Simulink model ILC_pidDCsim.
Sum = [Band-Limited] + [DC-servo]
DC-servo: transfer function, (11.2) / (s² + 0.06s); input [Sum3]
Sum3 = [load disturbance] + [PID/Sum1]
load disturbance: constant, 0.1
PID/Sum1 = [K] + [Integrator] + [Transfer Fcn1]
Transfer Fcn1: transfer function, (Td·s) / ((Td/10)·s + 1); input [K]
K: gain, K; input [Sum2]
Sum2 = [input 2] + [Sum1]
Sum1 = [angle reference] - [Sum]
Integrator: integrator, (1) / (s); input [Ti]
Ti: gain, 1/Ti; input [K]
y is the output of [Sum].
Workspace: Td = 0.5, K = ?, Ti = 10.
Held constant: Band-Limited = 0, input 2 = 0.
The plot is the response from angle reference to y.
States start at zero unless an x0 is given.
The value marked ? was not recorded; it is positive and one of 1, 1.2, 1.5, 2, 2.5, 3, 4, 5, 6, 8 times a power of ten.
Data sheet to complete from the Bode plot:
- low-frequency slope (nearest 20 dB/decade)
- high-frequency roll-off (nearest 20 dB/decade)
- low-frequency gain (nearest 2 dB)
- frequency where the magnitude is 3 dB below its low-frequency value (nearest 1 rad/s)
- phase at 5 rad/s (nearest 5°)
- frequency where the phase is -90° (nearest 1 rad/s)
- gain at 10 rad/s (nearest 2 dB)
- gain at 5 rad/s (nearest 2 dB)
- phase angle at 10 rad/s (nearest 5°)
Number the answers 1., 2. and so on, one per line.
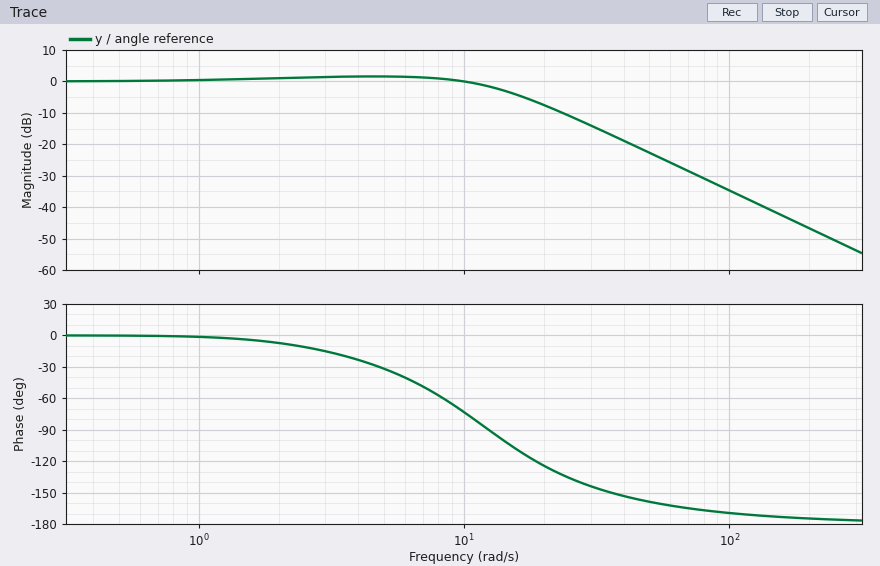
1. 0 dB/decade
2. -40 dB/decade
3. 0 dB
4. 14 rad/s
5. -30°
6. 12 rad/s
7. 0 dB
8. 2 dB
9. -75°
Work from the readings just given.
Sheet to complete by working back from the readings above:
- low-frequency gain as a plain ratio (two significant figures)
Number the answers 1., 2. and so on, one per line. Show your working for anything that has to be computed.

1. 10^(0 / 20) = 1.0
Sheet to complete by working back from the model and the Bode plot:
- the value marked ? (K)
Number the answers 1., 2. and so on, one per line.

1. 1.5
